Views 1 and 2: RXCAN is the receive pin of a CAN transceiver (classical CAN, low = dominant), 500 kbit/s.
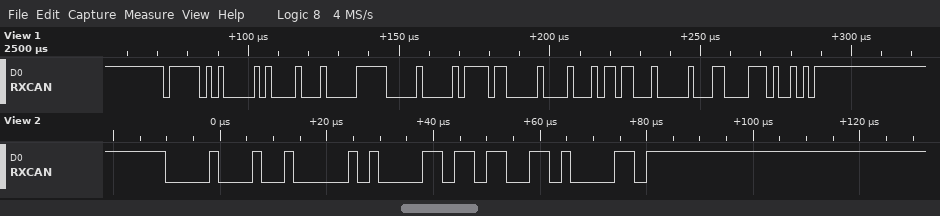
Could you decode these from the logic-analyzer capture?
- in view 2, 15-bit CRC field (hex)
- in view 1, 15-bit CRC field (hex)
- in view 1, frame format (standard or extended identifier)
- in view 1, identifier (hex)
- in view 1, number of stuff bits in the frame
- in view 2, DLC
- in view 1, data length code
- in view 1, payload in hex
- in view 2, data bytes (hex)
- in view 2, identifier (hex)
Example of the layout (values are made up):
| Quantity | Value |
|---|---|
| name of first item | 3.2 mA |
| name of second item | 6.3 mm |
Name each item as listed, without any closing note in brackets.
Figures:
| Quantity | Value |
|---|---|
| in view 2, 15-bit CRC field | 0x59A1 |
| in view 1, 15-bit CRC field | 0x61D2 |
| in view 1, frame format | standard |
| in view 1, identifier | 0x7E8 |
| in view 1, number of stuff bits in the frame | 8 |
| in view 2, DLC | 1 |
| in view 1, data length code | 8 |
| in view 1, payload in hex | 44 1E 00 7B 00 45 B1 00 |
| in view 2, data bytes | 0D |
| in view 2, identifier | 0x089 |
